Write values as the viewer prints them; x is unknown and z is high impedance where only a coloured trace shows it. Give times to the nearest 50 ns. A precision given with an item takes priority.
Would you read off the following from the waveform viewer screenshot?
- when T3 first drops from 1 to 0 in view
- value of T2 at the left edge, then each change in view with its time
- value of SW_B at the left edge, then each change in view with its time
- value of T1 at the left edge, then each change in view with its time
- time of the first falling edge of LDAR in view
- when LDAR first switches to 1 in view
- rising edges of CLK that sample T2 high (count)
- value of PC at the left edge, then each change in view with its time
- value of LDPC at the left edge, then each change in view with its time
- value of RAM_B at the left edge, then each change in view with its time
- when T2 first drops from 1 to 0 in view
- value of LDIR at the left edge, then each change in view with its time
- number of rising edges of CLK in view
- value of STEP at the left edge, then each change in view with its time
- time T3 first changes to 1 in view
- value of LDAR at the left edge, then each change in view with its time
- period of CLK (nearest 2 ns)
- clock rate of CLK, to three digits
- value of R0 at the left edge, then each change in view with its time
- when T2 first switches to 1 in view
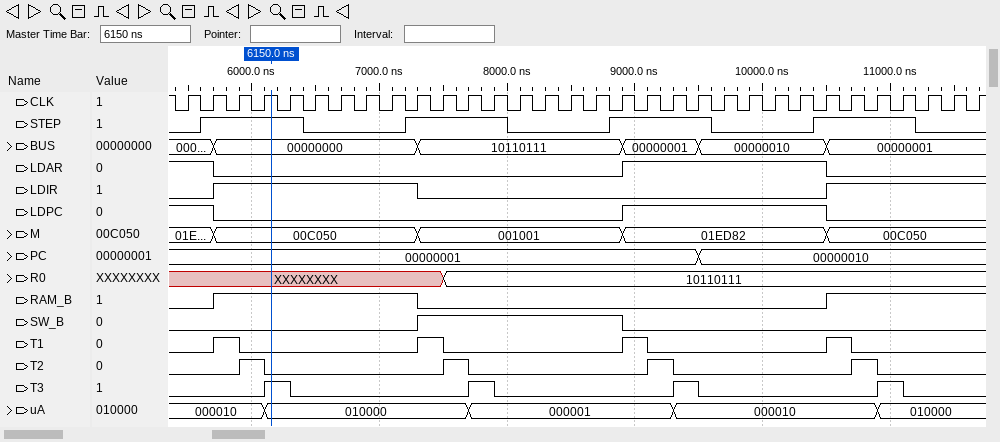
6300 ns
0, 1 at 5900 ns, 0 at 6100 ns, 1 at 7500 ns, 0 at 7700 ns, 1 at 9100 ns, 0 at 9300 ns, 1 at 10700 ns, 0 at 10900 ns
0, 1 at 7300 ns, 0 at 8900 ns
0, 1 at 5700 ns, 0 at 5900 ns, 1 at 7300 ns, 0 at 7500 ns, 1 at 8900 ns, 0 at 9100 ns, 1 at 10500 ns, 0 at 10700 ns
5700 ns
8900 ns
4
00000001, 00000010 at 9500 ns
1, 0 at 5700 ns, 1 at 8900 ns, 0 at 10500 ns
0, 1 at 5700 ns, 0 at 7300 ns, 1 at 10500 ns
6100 ns
0, 1 at 5700 ns, 0 at 7300 ns, 1 at 10500 ns
32
0, 1 at 5600 ns, 0 at 6400 ns, 1 at 7200 ns, 0 at 8000 ns, 1 at 8800 ns, 0 at 9600 ns, 1 at 10400 ns, 0 at 11200 ns
6100 ns
1, 0 at 5700 ns, 1 at 8900 ns, 0 at 10500 ns
200 ns
5.00 MHz
XXXXXXXX, 10110111 at 7500 ns
5900 ns
